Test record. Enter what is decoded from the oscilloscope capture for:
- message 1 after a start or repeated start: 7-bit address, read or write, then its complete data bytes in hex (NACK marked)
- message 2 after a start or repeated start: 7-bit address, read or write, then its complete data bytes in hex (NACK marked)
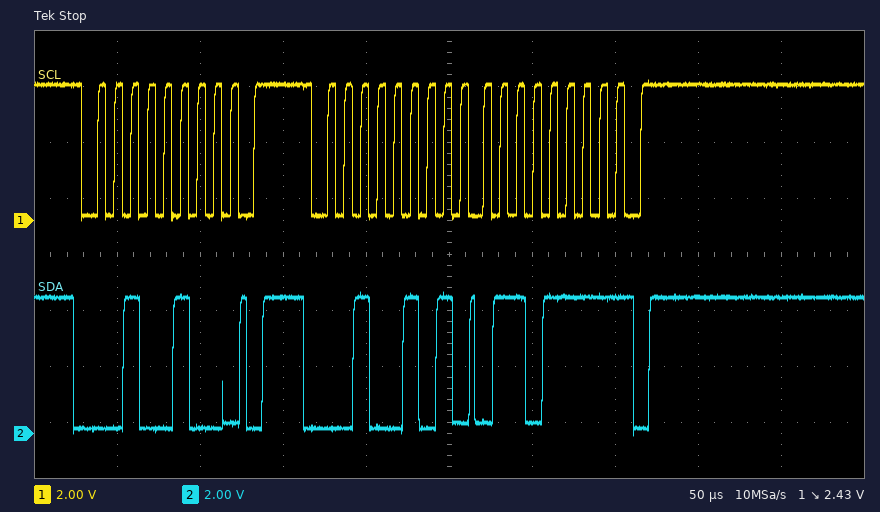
0x12 write
0x12 read: 6F NACK
